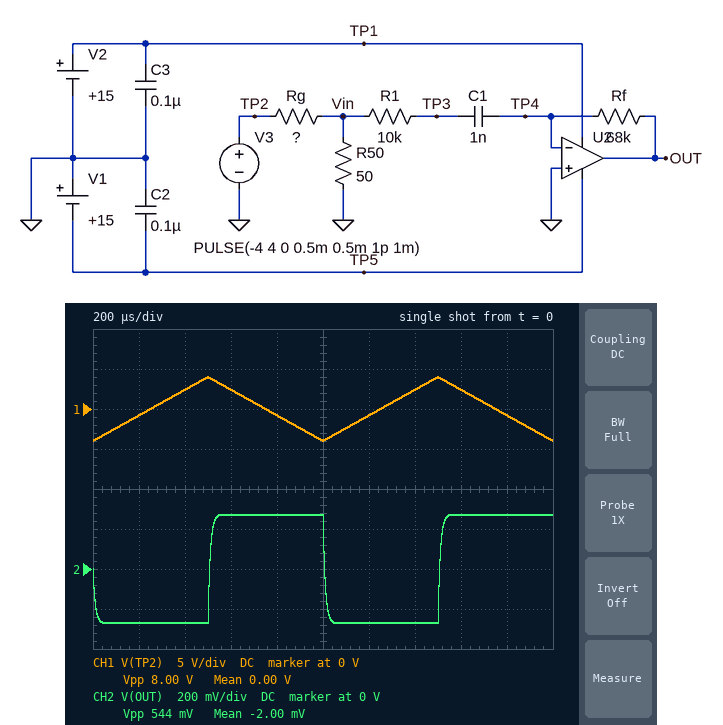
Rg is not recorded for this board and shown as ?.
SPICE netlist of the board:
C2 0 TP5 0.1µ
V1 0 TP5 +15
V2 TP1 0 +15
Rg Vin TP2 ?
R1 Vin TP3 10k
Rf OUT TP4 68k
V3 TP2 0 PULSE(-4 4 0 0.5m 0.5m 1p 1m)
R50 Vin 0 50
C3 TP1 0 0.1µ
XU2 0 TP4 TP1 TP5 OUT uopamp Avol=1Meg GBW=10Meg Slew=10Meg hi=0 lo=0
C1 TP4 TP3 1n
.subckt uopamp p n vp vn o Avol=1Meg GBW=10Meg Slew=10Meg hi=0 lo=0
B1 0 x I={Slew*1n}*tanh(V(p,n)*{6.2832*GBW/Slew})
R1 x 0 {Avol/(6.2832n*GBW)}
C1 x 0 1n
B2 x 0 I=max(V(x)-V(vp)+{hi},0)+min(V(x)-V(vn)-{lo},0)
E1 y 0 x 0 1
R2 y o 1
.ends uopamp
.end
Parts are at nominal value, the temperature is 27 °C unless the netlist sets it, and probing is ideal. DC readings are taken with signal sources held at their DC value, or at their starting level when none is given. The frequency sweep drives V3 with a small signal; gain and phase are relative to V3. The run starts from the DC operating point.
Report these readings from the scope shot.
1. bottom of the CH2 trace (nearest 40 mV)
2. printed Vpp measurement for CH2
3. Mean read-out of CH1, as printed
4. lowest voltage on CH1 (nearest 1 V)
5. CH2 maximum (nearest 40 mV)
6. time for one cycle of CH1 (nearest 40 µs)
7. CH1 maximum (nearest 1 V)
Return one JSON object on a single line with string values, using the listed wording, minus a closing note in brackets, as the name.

{"bottom of the CH2 trace": "-280 mV", "printed Vpp measurement for CH2": "544 mV", "Mean read-out of CH1, as printed": "0.00 V", "lowest voltage on CH1": "-4 V", "CH2 maximum": "280 mV", "time for one cycle of CH1": "1.00 ms", "CH1 maximum": "4 V"}
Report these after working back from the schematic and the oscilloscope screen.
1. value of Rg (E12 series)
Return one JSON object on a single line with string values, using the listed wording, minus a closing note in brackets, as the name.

{"value of Rg": "150 Ω"}
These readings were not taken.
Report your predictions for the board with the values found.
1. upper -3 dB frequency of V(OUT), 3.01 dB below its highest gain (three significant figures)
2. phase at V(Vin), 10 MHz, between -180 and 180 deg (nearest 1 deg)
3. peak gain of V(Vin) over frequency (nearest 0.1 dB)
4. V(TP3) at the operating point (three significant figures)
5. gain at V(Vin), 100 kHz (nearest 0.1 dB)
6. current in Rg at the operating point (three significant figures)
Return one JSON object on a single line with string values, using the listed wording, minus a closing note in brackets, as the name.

{"upper -3 dB frequency of V(OUT), 3.01 dB below its highest gain": "1.30 MHz", "phase at V(Vin), 10 MHz, between -180 and 180 deg": "0 deg", "peak gain of V(Vin) over frequency": "-12.0 dB", "V(TP3) at the operating point": "-1.00 V", "gain at V(Vin), 100 kHz": "-12.1 dB", "current in Rg at the operating point": "20.0 mA"}
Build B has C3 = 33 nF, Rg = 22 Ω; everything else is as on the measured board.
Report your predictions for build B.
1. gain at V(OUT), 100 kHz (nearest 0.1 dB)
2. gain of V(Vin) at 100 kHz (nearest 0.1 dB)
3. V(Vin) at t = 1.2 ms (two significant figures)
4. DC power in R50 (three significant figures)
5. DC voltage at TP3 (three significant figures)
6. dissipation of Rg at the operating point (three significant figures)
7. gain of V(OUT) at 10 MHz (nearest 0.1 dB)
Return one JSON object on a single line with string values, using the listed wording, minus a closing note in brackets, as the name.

{"gain at V(OUT), 100 kHz": "13.4 dB", "gain of V(Vin) at 100 kHz": "-3.2 dB", "V(Vin) at t = 1.2 ms": "-560 mV", "DC power in R50": "154 mW", "DC voltage at TP3": "-2.78 V", "dissipation of Rg at the operating point": "67.9 mW", "gain of V(OUT) at 10 MHz": "-4.4 dB"}
